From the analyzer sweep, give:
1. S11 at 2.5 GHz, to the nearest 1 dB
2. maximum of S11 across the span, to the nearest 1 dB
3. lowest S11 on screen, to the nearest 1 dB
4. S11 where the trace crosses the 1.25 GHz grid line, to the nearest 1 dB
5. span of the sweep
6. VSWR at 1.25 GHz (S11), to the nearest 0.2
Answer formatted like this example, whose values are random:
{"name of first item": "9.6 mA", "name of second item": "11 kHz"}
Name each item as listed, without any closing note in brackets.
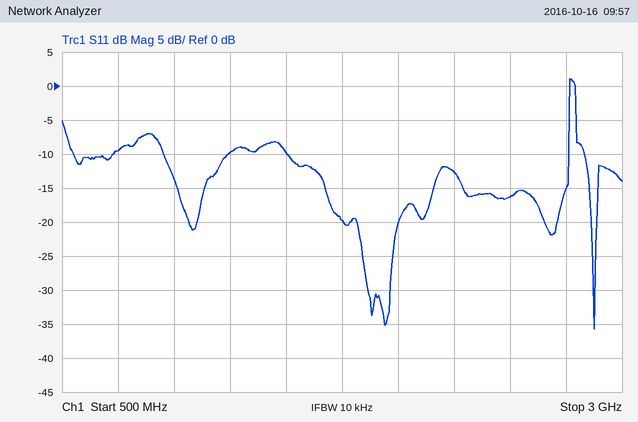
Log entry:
{"S11 at 2.5 GHz, to the nearest 1 dB": "-16 dB", "maximum of S11 across the span, to the nearest 1 dB": "1 dB", "lowest S11 on screen, to the nearest 1 dB": "-36 dB", "S11 where the trace crosses the 1.25 GHz grid line, to the nearest 1 dB": "-10 dB", "span of the sweep": "2.5 GHz", "VSWR at 1.25 GHz (S11), to the nearest 0.2": "2.0"}
